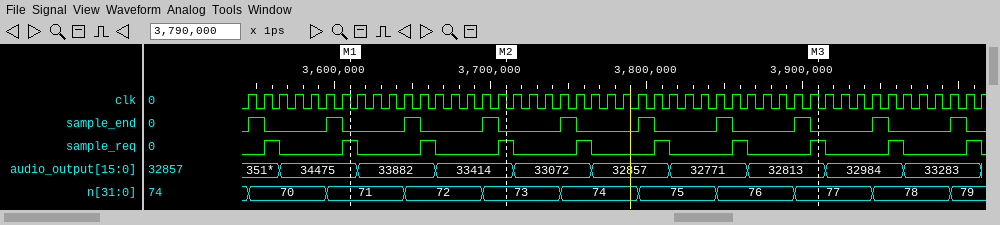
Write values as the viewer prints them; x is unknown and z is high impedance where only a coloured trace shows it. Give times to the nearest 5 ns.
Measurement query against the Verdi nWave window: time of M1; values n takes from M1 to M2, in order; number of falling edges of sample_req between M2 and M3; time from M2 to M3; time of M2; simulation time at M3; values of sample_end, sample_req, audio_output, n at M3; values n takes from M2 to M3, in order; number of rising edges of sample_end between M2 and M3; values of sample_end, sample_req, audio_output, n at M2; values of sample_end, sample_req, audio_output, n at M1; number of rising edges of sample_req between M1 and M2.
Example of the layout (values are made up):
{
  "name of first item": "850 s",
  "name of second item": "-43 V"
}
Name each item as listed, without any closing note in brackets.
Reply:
{
  "time of M1": "3610 ns",
  "values n takes from M1 to M2, in order": "71, 72, 73",
  "number of falling edges of sample_req between M2 and M3": "4",
  "time from M2 to M3": "200 ns",
  "time of M2": "3710 ns",
  "simulation time at M3": "3910 ns",
  "values of sample_end, sample_req, audio_output, n at M3": "sample_end=0, sample_req=1, audio_output=32813, n=77",
  "values n takes from M2 to M3, in order": "73, 74, 75, 76, 77",
  "number of rising edges of sample_end between M2 and M3": "4",
  "values of sample_end, sample_req, audio_output, n at M2": "sample_end=0, sample_req=1, audio_output=33414, n=73",
  "values of sample_end, sample_req, audio_output, n at M1": "sample_end=0, sample_req=1, audio_output=34475, n=71",
  "number of rising edges of sample_req between M1 and M2": "2"
}
